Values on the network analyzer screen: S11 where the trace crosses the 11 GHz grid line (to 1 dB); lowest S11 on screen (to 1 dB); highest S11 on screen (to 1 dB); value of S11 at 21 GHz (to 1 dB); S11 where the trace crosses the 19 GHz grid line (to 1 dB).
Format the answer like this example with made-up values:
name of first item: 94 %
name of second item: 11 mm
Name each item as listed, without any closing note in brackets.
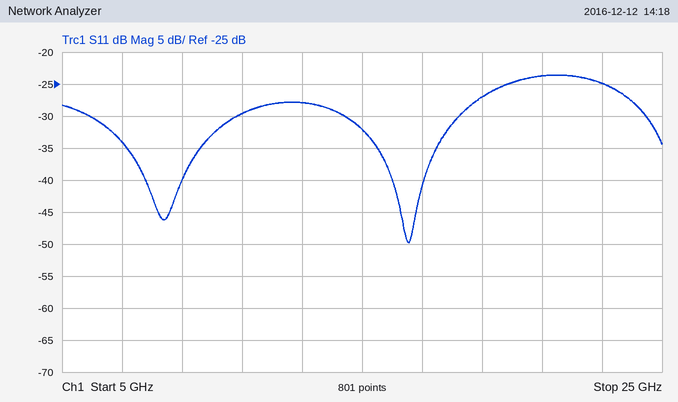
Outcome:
S11 where the trace crosses the 11 GHz grid line: -30 dB
lowest S11 on screen: -50 dB
highest S11 on screen: -24 dB
value of S11 at 21 GHz: -24 dB
S11 where the trace crosses the 19 GHz grid line: -27 dB
